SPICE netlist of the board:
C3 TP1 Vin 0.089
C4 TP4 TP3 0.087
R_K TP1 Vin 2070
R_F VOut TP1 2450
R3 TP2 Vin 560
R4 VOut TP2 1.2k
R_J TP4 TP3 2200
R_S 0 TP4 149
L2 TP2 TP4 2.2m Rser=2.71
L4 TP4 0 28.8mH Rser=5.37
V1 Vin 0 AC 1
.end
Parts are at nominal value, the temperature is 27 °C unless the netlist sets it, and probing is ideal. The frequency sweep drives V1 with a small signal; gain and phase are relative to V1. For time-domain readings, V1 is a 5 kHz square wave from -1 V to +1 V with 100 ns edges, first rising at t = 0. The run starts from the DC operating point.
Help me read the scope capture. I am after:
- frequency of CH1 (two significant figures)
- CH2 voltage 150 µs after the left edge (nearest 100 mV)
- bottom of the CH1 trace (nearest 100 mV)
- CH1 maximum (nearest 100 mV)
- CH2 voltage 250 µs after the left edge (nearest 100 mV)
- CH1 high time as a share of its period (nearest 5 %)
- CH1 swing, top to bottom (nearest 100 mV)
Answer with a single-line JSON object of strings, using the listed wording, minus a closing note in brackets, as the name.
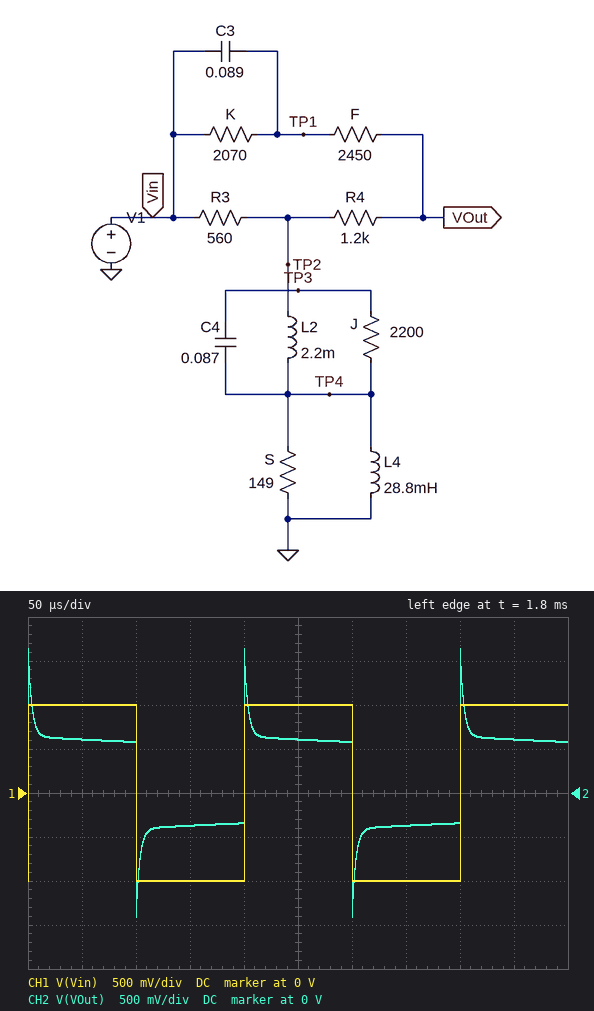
{"frequency of CH1": "5.0 kHz", "CH2 voltage 150 µs after the left edge": "-400 mV", "bottom of the CH1 trace": "-1.0 V", "CH1 maximum": "1.0 V", "CH2 voltage 250 µs after the left edge": "600 mV", "CH1 high time as a share of its period": "50 %", "CH1 swing, top to bottom": "2.0 V"}
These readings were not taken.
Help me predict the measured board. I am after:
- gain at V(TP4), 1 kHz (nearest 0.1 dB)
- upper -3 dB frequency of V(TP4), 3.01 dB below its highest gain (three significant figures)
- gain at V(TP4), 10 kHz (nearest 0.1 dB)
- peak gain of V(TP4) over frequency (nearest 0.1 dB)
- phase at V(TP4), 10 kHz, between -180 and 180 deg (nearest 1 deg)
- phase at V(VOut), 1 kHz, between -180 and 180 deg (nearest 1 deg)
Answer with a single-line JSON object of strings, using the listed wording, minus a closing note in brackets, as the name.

{"gain at V(TP4), 1 kHz": "-14.2 dB", "upper -3 dB frequency of V(TP4), 3.01 dB below its highest gain": "47.6 kHz", "gain at V(TP4), 10 kHz": "-12.9 dB", "peak gain of V(TP4) over frequency": "-12.8 dB", "phase at V(TP4), 10 kHz, between -180 and 180 deg": "-9 deg", "phase at V(VOut), 1 kHz, between -180 and 180 deg": "10 deg"}
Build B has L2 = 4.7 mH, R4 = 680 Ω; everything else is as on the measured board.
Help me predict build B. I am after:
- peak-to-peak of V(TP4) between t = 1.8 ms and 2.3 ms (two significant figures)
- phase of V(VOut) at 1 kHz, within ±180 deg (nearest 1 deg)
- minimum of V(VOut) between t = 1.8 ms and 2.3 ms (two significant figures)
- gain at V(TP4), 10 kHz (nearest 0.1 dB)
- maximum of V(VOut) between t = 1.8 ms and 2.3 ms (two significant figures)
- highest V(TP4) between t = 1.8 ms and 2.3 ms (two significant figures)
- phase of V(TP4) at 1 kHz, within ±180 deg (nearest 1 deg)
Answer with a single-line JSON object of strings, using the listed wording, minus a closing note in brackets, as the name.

{"peak-to-peak of V(TP4) between t = 1.8 ms and 2.3 ms": "500 mV", "phase of V(VOut) at 1 kHz, within ±180 deg": "17 deg", "minimum of V(VOut) between t = 1.8 ms and 2.3 ms": "-1.5 V", "gain at V(TP4), 10 kHz": "-13.4 dB", "maximum of V(VOut) between t = 1.8 ms and 2.3 ms": "1.7 V", "highest V(TP4) between t = 1.8 ms and 2.3 ms": "250 mV", "phase of V(TP4) at 1 kHz, within ±180 deg": "29 deg"}
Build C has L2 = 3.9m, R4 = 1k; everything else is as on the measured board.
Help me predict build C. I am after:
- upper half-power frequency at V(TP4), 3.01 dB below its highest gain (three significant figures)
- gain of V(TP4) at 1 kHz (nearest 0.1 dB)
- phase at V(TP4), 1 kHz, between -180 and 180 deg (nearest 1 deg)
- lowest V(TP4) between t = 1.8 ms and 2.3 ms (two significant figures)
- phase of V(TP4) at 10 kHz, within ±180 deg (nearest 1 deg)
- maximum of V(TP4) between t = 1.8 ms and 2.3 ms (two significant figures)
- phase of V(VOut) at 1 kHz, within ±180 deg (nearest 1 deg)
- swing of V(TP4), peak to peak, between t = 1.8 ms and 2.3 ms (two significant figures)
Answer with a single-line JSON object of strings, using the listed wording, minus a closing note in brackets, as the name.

{"upper half-power frequency at V(TP4), 3.01 dB below its highest gain": "27.3 kHz", "gain of V(TP4) at 1 kHz": "-14.2 dB", "phase at V(TP4), 1 kHz, between -180 and 180 deg": "29 deg", "lowest V(TP4) between t = 1.8 ms and 2.3 ms": "-250 mV", "phase of V(TP4) at 10 kHz, within ±180 deg": "-17 deg", "maximum of V(TP4) between t = 1.8 ms and 2.3 ms": "250 mV", "phase of V(VOut) at 1 kHz, within ±180 deg": "13 deg", "swing of V(TP4), peak to peak, between t = 1.8 ms and 2.3 ms": "500 mV"}
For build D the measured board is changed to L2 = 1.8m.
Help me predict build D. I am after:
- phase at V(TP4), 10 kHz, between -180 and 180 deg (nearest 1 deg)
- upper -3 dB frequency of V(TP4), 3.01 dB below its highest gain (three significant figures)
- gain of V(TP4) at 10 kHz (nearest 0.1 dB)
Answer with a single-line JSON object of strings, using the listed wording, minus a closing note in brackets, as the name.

{"phase at V(TP4), 10 kHz, between -180 and 180 deg": "-6 deg", "upper -3 dB frequency of V(TP4), 3.01 dB below its highest gain": "57.8 kHz", "gain of V(TP4) at 10 kHz": "-12.8 dB"}
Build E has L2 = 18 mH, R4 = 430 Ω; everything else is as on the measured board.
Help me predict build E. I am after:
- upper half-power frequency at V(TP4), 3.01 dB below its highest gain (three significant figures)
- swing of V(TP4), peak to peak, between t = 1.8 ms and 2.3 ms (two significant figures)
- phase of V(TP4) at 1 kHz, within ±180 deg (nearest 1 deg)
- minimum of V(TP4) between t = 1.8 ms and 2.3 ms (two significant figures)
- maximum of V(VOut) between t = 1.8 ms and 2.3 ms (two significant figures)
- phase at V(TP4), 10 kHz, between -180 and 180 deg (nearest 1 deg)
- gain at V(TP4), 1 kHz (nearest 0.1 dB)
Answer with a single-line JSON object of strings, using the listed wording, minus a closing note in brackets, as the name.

{"upper half-power frequency at V(TP4), 3.01 dB below its highest gain": "6.86 kHz", "swing of V(TP4), peak to peak, between t = 1.8 ms and 2.3 ms": "400 mV", "phase of V(TP4) at 1 kHz, within ±180 deg": "21 deg", "minimum of V(TP4) between t = 1.8 ms and 2.3 ms": "-200 mV", "maximum of V(VOut) between t = 1.8 ms and 2.3 ms": "1.7 V", "phase at V(TP4), 10 kHz, between -180 and 180 deg": "-57 deg", "gain at V(TP4), 1 kHz": "-14.3 dB"}
